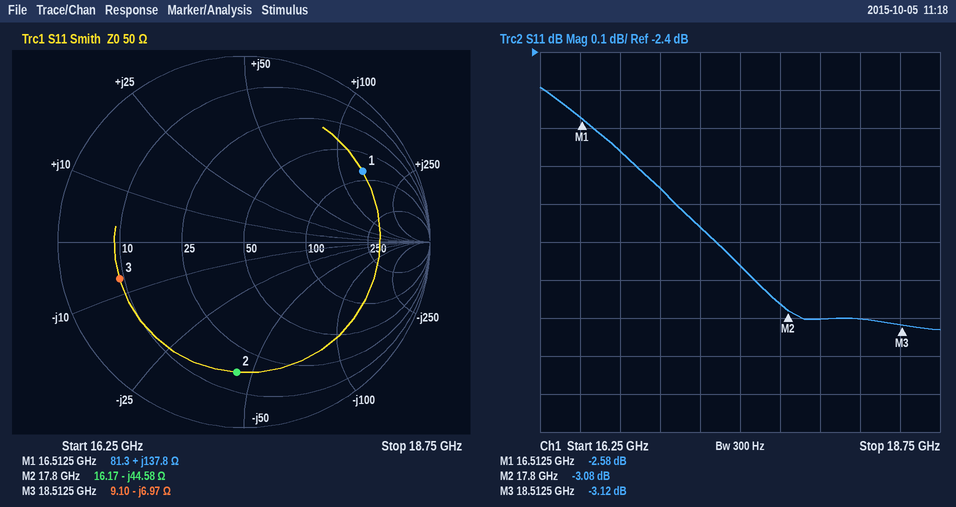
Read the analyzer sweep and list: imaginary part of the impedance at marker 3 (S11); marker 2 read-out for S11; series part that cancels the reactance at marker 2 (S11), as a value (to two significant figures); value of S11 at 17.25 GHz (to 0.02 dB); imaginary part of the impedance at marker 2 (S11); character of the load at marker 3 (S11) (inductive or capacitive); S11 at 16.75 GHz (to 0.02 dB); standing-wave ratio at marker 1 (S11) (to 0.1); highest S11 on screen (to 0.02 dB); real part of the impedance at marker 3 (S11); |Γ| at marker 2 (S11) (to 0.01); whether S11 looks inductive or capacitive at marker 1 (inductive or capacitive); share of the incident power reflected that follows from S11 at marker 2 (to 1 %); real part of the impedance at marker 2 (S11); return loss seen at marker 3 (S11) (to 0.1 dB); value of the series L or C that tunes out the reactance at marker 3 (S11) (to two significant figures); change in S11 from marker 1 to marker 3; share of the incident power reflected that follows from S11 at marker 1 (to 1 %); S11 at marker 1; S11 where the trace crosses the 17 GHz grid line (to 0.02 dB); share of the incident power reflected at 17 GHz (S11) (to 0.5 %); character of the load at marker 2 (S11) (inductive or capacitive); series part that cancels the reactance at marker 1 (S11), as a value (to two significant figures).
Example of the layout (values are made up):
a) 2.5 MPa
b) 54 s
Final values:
a) -6.97 Ω
b) -3.08 dB
c) 400 pH
d) -2.86 dB
e) -44.58 Ω
f) capacitive
g) -2.66 dB
h) 6.8
i) -2.50 dB
j) 9.10 Ω
k) 0.70
l) inductive
m) 49 %
n) 16.17 Ω
o) 3.1 dB
p) 60 pH
q) -0.54 dB
r) 55 %
s) -2.58 dB
t) -2.76 dB
u) 53.0 %
v) capacitive
w) 70 fF
